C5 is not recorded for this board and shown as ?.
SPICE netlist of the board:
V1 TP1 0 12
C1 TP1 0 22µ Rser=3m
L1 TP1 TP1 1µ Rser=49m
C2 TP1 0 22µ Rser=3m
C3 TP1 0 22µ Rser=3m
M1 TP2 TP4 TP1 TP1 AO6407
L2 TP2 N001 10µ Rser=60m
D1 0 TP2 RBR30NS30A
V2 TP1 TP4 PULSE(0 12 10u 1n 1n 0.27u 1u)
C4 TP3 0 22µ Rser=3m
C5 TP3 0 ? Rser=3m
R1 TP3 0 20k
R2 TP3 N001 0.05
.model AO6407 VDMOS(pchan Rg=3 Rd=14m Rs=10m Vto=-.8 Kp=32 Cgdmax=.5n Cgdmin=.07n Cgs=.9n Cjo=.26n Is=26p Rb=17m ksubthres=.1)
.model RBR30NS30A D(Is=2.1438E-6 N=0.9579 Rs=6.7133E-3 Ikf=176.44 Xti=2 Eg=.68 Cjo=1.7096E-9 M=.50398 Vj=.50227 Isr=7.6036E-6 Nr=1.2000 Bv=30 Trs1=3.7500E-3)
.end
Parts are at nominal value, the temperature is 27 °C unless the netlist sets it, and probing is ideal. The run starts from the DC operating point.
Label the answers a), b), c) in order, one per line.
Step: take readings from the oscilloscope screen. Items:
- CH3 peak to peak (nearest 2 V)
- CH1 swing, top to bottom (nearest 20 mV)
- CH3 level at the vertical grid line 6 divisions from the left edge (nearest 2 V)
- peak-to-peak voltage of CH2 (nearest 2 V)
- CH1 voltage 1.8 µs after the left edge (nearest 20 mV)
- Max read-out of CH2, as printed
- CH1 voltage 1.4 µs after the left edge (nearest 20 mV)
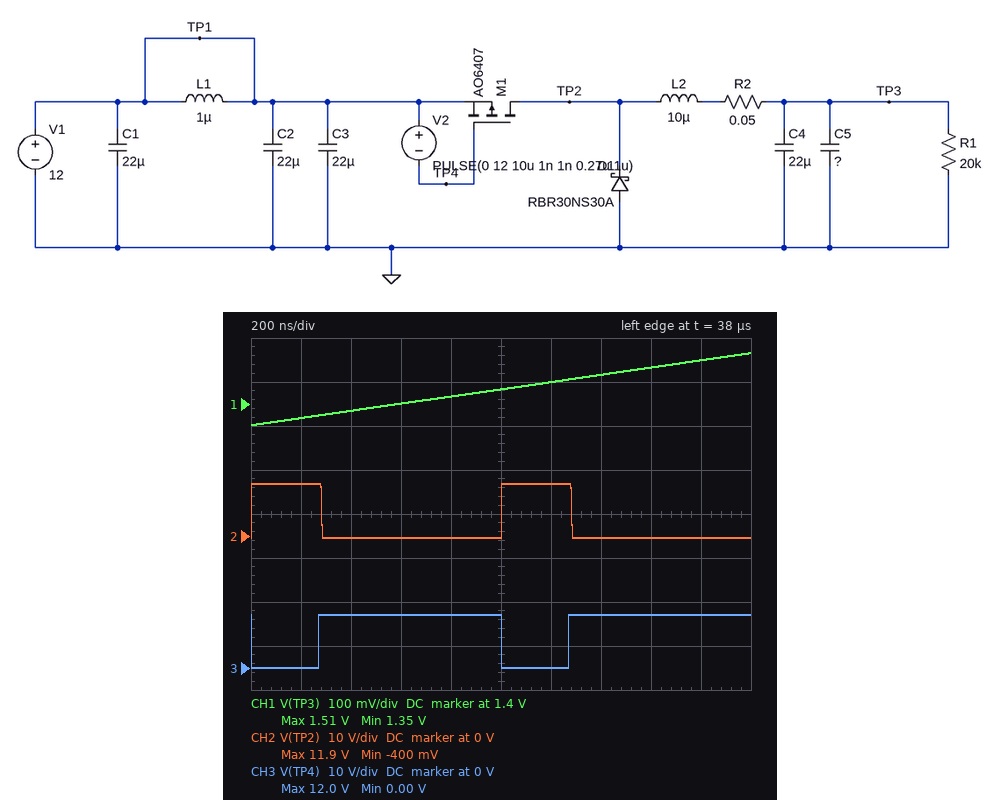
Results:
a) 12 V
b) 160 mV
c) 0 V
d) 12 V
e) 1.50 V
f) 11.9 V
g) 1.46 V
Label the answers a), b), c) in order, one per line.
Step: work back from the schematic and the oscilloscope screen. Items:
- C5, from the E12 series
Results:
a) 56 µF
